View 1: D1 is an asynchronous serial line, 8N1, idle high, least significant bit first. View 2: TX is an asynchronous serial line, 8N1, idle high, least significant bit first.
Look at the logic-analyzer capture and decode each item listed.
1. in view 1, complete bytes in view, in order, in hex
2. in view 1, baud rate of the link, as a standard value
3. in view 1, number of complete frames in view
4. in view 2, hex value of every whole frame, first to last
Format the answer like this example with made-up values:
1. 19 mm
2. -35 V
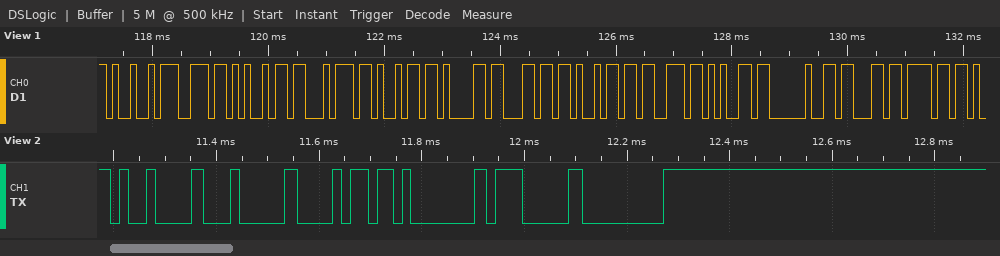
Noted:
1. 49 6E 69 74 69 61 6C 69 73 65 20 63 6F
2. 9600 baud
3. 13
4. 0x09 0x04 0x68 0x01 0x07 0x00
